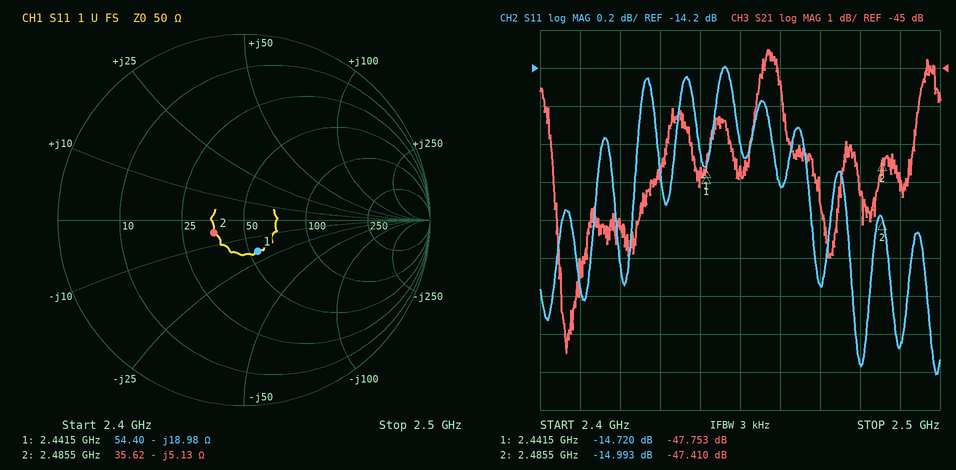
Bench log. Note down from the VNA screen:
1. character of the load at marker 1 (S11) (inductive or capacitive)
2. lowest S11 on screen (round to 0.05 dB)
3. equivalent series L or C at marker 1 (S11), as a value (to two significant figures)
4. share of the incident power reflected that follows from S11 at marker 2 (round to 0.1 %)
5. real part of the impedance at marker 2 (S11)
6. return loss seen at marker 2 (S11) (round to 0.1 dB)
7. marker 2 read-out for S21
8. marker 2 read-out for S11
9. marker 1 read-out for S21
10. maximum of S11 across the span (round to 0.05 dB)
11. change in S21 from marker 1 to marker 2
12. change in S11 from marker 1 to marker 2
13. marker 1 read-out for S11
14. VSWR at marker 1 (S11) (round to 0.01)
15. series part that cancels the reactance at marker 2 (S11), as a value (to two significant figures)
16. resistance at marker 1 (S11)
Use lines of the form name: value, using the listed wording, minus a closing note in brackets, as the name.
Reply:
character of the load at marker 1 (S11): capacitive
lowest S11 on screen: -15.80 dB
equivalent series L or C at marker 1 (S11), as a value: 3.4 pF
share of the incident power reflected that follows from S11 at marker 2: 3.2 %
real part of the impedance at marker 2: 35.62 Ω
return loss seen at marker 2 (S11): 15.0 dB
marker 2 read-out for S21: -47.410 dB
marker 2 read-out for S11: -14.993 dB
marker 1 read-out for S21: -47.753 dB
maximum of S11 across the span: -14.20 dB
change in S21 from marker 1 to marker 2: 0.343 dB
change in S11 from marker 1 to marker 2: -0.273 dB
marker 1 read-out for S11: -14.720 dB
VSWR at marker 1 (S11): 1.45
series part that cancels the reactance at marker 2 (S11), as a value: 330 pH
resistance at marker 1: 54.40 Ω
